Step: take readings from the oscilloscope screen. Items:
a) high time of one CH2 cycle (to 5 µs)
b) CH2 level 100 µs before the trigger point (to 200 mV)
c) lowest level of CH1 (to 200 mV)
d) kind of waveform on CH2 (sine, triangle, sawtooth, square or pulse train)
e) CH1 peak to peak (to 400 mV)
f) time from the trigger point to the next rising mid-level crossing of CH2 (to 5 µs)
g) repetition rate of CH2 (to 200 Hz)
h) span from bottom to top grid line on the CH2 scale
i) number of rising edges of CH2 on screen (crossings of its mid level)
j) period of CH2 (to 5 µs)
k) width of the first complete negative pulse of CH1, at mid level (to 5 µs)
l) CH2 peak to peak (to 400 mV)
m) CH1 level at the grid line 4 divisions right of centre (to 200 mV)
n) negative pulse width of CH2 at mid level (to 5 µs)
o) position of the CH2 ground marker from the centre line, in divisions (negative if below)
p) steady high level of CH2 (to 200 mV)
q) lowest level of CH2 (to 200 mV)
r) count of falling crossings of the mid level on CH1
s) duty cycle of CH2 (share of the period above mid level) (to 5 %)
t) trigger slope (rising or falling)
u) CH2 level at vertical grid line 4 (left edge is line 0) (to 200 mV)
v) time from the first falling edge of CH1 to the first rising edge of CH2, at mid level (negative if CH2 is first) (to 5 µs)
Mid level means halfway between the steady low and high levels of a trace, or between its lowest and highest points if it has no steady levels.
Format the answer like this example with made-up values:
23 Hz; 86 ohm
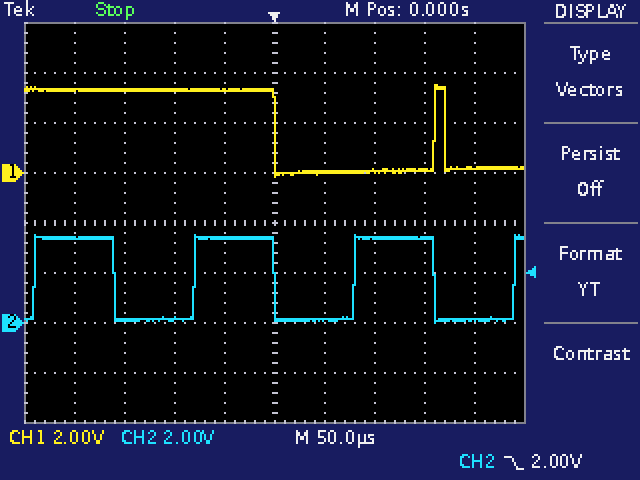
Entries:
80 µs; 200 mV; -200 mV; square; 3.6 V; 80 µs; 6.2 kHz; 16 V; 4; 160 µs; 160 µs; 3.6 V; 200 mV; 80 µs; -2.0 div; 3.4 V; 0.0 V; 2; 50 %; falling; 3.4 V; -240 µs
